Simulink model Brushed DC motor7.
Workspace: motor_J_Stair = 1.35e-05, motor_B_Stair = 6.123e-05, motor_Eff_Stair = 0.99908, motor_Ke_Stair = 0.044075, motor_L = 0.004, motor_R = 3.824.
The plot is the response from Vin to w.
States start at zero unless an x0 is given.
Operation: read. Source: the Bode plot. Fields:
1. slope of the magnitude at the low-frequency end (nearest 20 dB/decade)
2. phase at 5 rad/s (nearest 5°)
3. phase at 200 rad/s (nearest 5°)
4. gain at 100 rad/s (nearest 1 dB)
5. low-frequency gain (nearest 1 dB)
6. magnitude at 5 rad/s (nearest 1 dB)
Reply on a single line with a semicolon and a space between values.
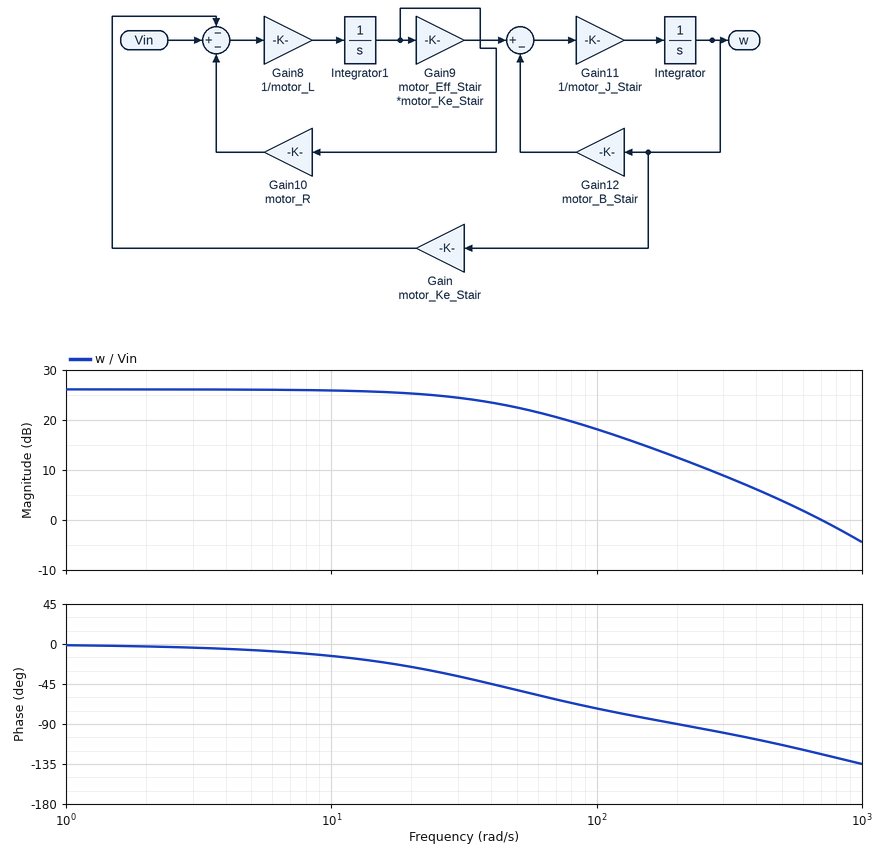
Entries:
0 dB/decade; -5°; -90°; 18 dB; 26 dB; 26 dB
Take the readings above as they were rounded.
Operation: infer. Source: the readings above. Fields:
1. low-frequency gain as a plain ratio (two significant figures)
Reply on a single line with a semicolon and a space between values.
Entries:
20
